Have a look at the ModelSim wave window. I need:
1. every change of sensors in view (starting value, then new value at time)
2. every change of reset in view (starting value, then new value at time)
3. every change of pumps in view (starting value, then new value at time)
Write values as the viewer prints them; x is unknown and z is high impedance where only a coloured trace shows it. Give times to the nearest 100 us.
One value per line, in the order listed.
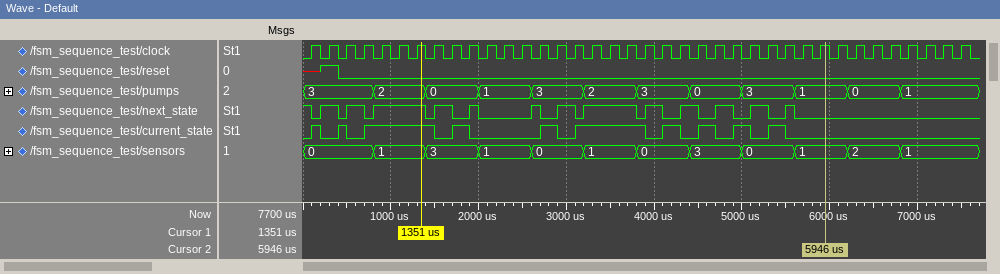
0, 1 at 800 us, 3 at 1400 us, 1 at 2000 us, 0 at 2600 us, 1 at 3200 us, 0 at 3800 us, 3 at 4400 us, 0 at 5000 us, 1 at 5600 us, 2 at 6200 us, 1 at 6800 us
x, 1 at 200 us, 0 at 400 us
3, 2 at 800 us, 0 at 1400 us, 1 at 2000 us, 3 at 2600 us, 2 at 3200 us, 3 at 3800 us, 0 at 4400 us, 3 at 5000 us, 1 at 5600 us, 0 at 6200 us, 1 at 6800 us
